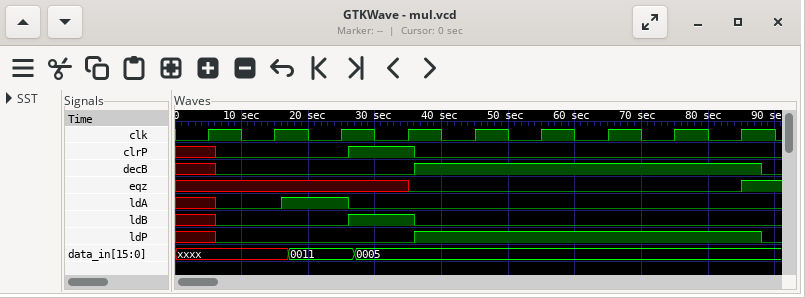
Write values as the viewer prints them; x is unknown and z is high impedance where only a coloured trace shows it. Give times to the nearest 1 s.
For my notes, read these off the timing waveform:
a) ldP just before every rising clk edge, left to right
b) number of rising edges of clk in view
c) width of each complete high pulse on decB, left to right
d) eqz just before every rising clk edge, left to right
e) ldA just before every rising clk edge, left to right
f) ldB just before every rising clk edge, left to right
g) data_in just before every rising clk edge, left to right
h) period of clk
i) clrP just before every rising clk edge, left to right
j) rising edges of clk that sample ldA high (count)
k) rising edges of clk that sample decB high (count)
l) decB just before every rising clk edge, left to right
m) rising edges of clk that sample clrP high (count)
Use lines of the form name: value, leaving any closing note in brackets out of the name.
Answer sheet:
ldP just before every rising clk edge, left to right: x 0 0 0 1 1 1 1 1
number of rising edges of clk in view: 9
width of each complete high pulse on decB, left to right: 52 s
eqz just before every rising clk edge, left to right: x x x x 0 0 0 0 0
ldA just before every rising clk edge, left to right: x 0 1 0 0 0 0 0 0
ldB just before every rising clk edge, left to right: x 0 0 1 0 0 0 0 0
data_in just before every rising clk edge, left to right: xxxx, xxxx, 0011, 0005, 0005, 0005, 0005, 0005, 0005
period of clk: 10 s
clrP just before every rising clk edge, left to right: x 0 0 1 0 0 0 0 0
rising edges of clk that sample ldA high: 1
rising edges of clk that sample decB high: 5
decB just before every rising clk edge, left to right: x 0 0 0 1 1 1 1 1
rising edges of clk that sample clrP high: 1
